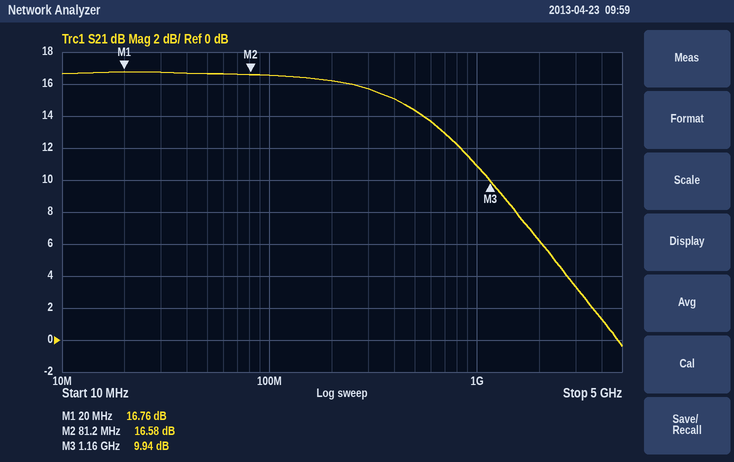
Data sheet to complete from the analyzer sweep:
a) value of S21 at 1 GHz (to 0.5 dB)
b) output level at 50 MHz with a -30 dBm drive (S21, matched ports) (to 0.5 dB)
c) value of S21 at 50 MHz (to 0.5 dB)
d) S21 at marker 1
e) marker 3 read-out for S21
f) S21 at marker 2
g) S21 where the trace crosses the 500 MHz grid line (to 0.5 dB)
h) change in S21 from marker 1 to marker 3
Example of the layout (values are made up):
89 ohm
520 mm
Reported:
11.0 dB
-13.5 dBm
16.5 dB
16.76 dB
9.94 dB
16.58 dB
14.5 dB
-6.82 dB
